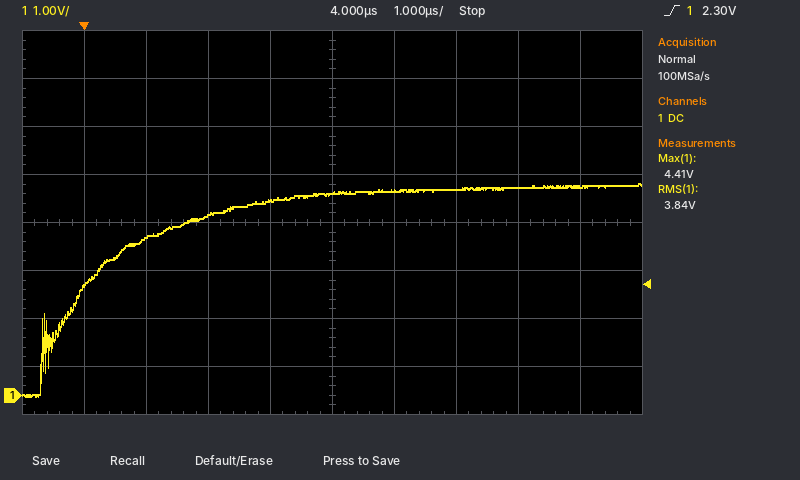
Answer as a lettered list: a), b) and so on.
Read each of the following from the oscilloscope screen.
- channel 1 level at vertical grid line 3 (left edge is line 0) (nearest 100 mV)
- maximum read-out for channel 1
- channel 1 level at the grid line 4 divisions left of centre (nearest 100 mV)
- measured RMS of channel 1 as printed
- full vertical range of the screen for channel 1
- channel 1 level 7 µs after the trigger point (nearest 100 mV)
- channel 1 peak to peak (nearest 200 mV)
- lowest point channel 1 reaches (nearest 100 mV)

a) 3.8 V
b) 4.41 V
c) 2.3 V
d) 3.84 V
e) 8 V
f) 4.3 V
g) 4.4 V
h) 0.0 V
